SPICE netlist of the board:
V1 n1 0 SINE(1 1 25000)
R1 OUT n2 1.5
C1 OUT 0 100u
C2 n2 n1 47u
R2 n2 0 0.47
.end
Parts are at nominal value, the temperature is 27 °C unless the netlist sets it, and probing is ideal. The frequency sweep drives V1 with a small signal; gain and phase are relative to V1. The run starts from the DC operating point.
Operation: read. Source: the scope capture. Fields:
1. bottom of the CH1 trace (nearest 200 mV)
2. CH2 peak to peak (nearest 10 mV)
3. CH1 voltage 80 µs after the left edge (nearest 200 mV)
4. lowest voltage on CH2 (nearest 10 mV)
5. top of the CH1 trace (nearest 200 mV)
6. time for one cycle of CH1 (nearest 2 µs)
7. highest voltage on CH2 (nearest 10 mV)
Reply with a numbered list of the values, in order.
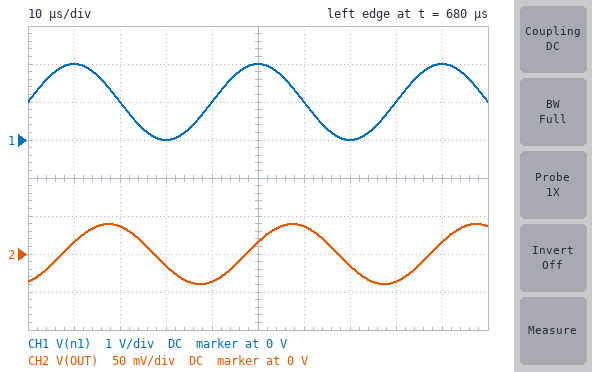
1. 0 V
2. 80 mV
3. 1.0 V
4. -40 mV
5. 2.0 V
6. 40 µs
7. 40 mV
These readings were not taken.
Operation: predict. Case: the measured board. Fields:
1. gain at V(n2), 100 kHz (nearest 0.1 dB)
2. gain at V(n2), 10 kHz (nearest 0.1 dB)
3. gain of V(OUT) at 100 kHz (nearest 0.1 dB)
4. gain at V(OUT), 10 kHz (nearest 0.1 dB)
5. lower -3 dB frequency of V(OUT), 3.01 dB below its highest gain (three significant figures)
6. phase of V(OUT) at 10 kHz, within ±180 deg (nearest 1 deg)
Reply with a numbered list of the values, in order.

1. 0 dB
2. -2.9 dB
3. -39.5 dB
4. -22.4 dB
5. 682 Hz
6. -41 deg
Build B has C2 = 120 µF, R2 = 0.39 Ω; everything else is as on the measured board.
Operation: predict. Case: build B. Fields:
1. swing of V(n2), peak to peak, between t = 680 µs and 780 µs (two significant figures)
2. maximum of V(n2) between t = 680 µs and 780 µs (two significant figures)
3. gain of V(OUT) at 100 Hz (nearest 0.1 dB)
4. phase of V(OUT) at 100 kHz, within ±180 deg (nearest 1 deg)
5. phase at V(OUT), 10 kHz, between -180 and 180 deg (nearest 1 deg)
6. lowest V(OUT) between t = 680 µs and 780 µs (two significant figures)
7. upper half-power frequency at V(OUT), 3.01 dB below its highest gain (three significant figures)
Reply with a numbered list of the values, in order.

1. 2.0 V
2. 980 mV
3. -30.7 dB
4. -87 deg
5. -61 deg
6. -42 mV
7. 5.95 kHz
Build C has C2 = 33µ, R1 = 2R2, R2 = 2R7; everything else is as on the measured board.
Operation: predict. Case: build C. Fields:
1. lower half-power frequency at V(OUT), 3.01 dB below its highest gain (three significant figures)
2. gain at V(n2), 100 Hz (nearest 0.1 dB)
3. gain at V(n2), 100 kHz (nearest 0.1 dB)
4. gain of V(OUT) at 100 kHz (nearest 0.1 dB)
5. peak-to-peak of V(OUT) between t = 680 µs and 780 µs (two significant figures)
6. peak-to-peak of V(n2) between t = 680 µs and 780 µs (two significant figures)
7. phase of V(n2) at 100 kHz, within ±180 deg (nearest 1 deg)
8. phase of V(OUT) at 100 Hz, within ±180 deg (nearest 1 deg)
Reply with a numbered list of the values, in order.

1. 260 Hz
2. -25.4 dB
3. 0 dB
4. -42.8 dB
5. 57 mV
6. 2.0 V
7. 2 deg
8. 70 deg
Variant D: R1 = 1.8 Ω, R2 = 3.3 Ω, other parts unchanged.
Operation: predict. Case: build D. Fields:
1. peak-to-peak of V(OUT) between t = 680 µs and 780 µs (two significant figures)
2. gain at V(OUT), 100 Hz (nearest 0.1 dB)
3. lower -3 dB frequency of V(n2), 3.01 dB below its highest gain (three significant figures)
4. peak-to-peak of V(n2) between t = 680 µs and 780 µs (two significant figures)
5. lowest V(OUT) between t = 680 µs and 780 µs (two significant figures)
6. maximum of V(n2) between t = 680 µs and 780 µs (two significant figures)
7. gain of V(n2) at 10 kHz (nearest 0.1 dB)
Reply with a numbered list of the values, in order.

1. 70 mV
2. -20.8 dB
3. 3.33 kHz
4. 2.0 V
5. -36 mV
6. 990 mV
7. -0.5 dB
